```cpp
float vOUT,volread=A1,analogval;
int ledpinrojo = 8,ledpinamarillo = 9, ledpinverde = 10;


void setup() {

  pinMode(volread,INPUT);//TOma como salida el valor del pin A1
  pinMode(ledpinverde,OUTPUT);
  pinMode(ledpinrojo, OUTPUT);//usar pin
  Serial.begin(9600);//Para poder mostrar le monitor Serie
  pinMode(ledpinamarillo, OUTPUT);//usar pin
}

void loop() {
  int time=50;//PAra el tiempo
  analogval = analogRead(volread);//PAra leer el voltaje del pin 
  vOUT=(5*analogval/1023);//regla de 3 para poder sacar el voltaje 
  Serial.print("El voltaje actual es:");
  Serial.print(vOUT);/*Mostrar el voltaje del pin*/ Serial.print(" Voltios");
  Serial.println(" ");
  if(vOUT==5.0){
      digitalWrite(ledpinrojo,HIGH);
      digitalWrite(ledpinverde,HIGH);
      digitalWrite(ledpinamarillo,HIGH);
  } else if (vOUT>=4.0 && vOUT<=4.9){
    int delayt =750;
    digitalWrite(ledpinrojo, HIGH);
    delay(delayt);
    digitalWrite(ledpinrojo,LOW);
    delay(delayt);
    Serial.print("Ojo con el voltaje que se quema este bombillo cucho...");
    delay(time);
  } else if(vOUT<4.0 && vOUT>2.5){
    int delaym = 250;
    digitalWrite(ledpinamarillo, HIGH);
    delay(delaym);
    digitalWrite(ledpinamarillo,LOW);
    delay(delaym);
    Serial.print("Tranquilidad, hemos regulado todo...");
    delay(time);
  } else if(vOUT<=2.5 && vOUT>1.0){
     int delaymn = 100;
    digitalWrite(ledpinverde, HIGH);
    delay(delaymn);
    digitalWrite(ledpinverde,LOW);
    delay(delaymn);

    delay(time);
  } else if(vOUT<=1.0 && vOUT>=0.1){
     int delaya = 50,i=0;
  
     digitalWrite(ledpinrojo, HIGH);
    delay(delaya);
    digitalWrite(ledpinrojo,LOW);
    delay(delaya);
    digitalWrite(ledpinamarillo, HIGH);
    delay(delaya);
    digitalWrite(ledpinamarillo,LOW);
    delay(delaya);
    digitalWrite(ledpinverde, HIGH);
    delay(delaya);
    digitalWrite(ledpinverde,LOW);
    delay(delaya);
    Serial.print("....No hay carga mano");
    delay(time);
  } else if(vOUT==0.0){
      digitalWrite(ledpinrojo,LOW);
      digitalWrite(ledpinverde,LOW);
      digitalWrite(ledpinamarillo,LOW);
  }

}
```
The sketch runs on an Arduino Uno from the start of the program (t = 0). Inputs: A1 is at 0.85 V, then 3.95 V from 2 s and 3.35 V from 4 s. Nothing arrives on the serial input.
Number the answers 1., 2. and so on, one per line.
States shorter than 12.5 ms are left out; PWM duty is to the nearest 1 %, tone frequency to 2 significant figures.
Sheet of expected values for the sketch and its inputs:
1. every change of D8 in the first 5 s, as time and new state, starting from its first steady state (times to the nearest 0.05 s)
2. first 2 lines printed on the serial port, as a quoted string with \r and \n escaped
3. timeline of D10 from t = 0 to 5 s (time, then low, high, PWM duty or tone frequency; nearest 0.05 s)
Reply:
1. 0 s high; 0.05 s low; 0.35 s high; 0.4 s low; 0.7 s high; 0.75 s low; 1.05 s high; 1.1 s low; 1.4 s high; 1.45 s low; 1.75 s high; 1.8 s low
2. "El voltaje actual es:0.85 Voltios \r\n....No hay carga manoEl voltaje actual es:0.85 Voltios \r\n"
3. 0 s low; 0.2 s high; 0.25 s low; 0.55 s high; 0.6 s low; 0.9 s high; 0.95 s low; 1.25 s high; 1.3 s low; 1.6 s high; 1.65 s low; 1.95 s high; 2 s low
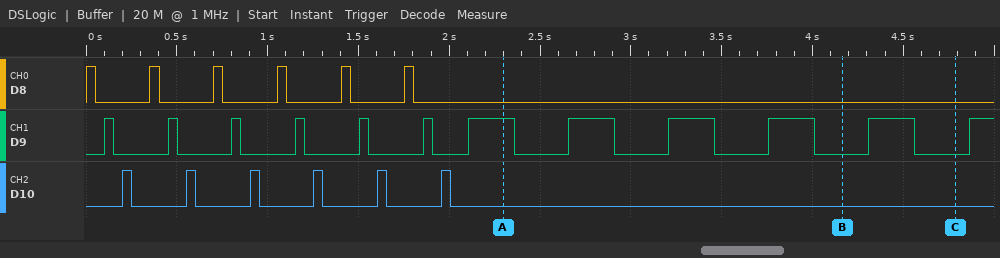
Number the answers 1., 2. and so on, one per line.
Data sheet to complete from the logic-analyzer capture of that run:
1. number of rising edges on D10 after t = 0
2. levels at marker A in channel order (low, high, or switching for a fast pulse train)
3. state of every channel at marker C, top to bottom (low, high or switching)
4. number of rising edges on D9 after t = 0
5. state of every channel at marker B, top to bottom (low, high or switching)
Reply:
1. 6
2. D8 low, D9 high, D10 low
3. D8 low, D9 low, D10 low
4. 12
5. D8 low, D9 low, D10 low
